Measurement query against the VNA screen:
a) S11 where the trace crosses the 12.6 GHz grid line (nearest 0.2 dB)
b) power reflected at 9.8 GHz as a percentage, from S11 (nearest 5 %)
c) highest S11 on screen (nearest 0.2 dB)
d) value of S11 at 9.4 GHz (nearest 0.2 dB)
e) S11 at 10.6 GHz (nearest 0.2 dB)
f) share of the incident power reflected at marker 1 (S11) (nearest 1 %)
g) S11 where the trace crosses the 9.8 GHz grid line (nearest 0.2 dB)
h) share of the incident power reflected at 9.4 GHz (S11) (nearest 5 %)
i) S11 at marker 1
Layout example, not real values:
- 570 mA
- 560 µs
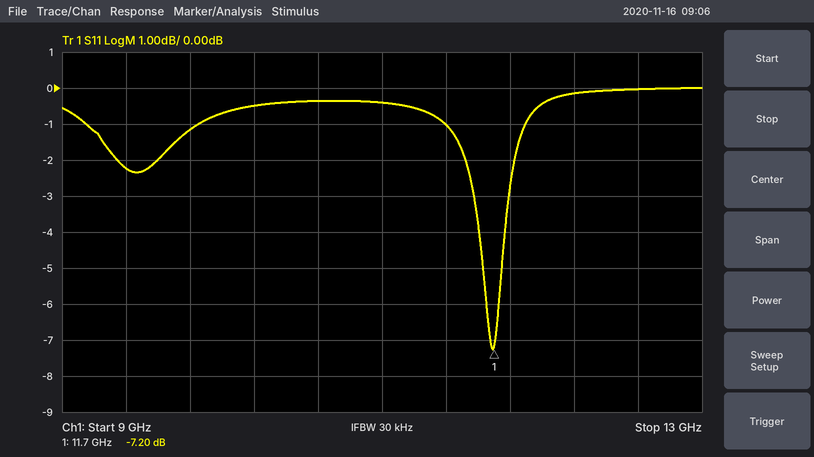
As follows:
- 0.0 dB
- 75 %
- 0.0 dB
- -2.2 dB
- -0.4 dB
- 19 %
- -1.2 dB
- 60 %
- -7.20 dB
